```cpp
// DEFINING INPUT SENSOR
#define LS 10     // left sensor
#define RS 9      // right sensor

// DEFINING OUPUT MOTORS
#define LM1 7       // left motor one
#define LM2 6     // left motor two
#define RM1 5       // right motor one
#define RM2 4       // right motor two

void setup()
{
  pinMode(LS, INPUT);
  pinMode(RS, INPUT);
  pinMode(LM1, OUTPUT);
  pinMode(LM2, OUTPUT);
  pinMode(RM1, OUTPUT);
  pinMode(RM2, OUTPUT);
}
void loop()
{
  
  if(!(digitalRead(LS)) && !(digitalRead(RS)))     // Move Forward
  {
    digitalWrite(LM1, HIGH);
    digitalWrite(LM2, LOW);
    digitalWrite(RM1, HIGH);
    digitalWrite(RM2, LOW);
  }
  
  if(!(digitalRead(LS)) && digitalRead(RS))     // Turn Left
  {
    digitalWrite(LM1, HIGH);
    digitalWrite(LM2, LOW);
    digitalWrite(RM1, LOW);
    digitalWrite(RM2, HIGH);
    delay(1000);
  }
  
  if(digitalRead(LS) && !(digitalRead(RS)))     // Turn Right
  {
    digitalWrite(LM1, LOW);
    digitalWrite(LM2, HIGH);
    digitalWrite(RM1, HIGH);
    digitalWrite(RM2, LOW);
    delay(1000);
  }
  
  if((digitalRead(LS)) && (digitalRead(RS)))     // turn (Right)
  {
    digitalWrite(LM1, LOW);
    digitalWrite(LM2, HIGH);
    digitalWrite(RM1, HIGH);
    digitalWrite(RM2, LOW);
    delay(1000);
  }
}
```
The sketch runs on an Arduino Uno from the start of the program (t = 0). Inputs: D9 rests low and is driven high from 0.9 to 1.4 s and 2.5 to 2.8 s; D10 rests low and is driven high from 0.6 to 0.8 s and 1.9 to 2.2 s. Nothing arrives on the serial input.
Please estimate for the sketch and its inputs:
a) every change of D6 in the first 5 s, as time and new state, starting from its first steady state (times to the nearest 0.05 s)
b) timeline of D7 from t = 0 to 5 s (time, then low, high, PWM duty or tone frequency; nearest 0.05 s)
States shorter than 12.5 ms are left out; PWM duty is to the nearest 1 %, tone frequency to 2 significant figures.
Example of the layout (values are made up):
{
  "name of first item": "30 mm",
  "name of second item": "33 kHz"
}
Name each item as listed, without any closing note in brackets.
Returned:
{
  "every change of D6 in the first 5 s, as time and new state, starting from its first steady state": "0 s low; 0.6 s high; 1.6 s low; 1.9 s high; 2.9 s low",
  "timeline of D7 from t = 0 to 5 s": "0 s high; 0.6 s low; 1.6 s high; 1.9 s low; 2.9 s high"
}
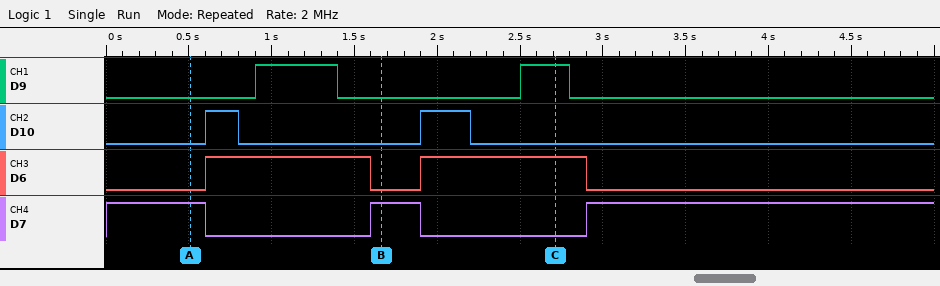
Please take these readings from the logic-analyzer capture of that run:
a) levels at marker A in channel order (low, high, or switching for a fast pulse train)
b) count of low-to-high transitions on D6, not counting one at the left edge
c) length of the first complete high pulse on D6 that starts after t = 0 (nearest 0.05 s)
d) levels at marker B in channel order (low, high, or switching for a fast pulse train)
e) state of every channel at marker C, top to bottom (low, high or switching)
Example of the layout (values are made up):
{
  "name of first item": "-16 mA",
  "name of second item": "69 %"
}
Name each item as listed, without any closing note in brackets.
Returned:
{
  "levels at marker A in channel order": "D9 low, D10 low, D6 low, D7 high",
  "count of low-to-high transitions on D6, not counting one at the left edge": "2",
  "length of the first complete high pulse on D6 that starts after t = 0": "1.00 s",
  "levels at marker B in channel order": "D9 low, D10 low, D6 low, D7 high",
  "state of every channel at marker C, top to bottom": "D9 high, D10 low, D6 high, D7 low"
}
